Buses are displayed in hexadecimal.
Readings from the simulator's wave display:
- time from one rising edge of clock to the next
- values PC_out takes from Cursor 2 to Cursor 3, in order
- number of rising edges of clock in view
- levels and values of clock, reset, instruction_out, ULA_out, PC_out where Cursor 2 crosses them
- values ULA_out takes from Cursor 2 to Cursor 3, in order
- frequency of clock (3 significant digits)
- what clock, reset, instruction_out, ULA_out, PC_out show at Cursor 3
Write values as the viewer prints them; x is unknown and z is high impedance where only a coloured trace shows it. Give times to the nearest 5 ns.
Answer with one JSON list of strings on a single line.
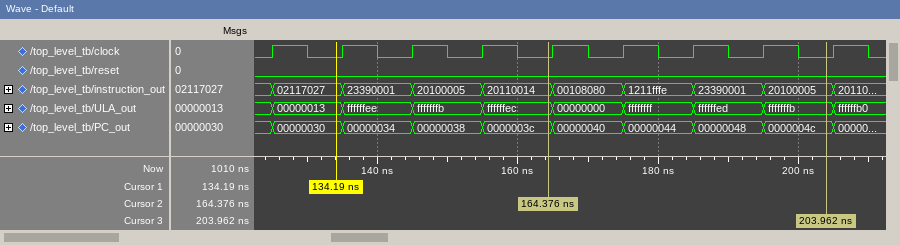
["10 ns", "0000003c, 00000040, 00000044, 00000048, 0000004c", "9", "clock=0, reset=0, instruction_out=20110014, ULA_out=ffffffec, PC_out=0000003c", "ffffffec, 00000000, ffffffff, ffffffed, fffffffb", "100 MHz", "clock=0, reset=0, instruction_out=20100005, ULA_out=fffffffb, PC_out=0000004c"]
